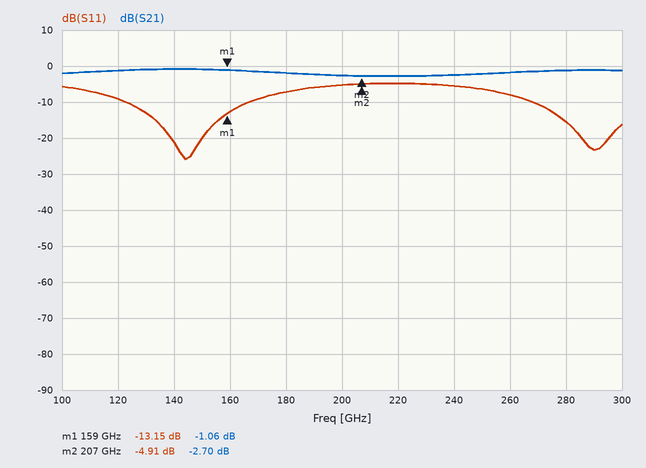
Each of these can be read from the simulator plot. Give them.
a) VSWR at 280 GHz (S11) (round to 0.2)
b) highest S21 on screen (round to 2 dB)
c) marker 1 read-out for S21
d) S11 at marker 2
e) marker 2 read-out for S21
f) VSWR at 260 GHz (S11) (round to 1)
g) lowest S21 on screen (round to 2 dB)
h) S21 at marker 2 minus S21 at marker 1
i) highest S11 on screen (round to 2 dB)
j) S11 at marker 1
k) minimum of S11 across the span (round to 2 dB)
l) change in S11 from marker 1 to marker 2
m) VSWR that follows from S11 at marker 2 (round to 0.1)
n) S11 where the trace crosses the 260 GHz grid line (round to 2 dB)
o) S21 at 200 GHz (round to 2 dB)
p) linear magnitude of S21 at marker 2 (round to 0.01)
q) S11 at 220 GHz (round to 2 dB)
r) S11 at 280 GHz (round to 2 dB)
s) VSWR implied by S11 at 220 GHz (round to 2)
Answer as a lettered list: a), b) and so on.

a) 1.4
b) 0 dB
c) -1.06 dB
d) -4.91 dB
e) -2.70 dB
f) 2
g) -2 dB
h) -1.64 dB
i) -4 dB
j) -13.15 dB
k) -26 dB
l) 8.24 dB
m) 3.6
n) -8 dB
o) -2 dB
p) 0.73
q) -4 dB
r) -16 dB
s) 4
